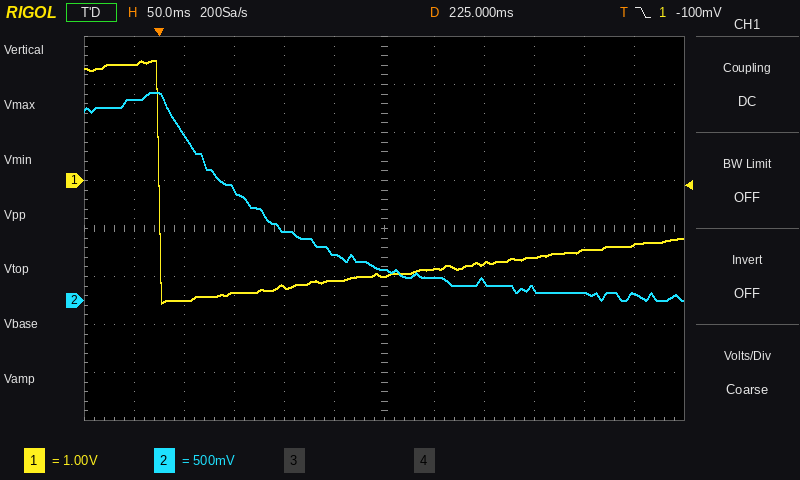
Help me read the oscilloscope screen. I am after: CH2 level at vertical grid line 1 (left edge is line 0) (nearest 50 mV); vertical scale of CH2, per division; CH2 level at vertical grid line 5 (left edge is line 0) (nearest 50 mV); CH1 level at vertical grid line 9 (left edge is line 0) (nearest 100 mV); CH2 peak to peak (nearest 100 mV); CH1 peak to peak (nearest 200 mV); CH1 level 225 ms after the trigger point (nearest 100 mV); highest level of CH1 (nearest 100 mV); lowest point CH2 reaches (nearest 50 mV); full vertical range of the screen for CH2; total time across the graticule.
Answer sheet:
2.10 V
500 mV
500 mV
-1.6 V
2.20 V
5.0 V
-2.0 V
2.5 V
0 mV
4 V
600 ms
